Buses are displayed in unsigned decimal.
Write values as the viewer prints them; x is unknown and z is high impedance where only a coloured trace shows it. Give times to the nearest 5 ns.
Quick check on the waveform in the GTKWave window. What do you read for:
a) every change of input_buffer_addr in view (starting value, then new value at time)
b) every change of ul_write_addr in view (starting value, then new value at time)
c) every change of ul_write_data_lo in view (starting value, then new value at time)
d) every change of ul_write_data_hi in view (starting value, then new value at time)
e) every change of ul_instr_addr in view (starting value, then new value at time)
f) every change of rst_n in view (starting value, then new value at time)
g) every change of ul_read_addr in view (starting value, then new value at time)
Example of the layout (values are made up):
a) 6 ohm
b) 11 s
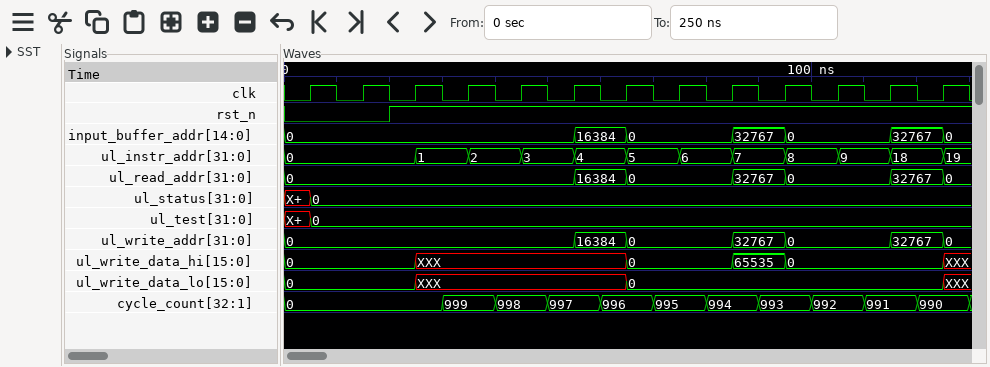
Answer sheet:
a) 0, 16384 at 55 ns, 0 at 65 ns, 32767 at 85 ns, 0 at 95 ns, 32767 at 115 ns, 0 at 125 ns
b) 0, 16384 at 55 ns, 0 at 65 ns, 32767 at 85 ns, 0 at 95 ns, 32767 at 115 ns, 0 at 125 ns
c) 0, XXX at 25 ns, 0 at 65 ns, XXX at 125 ns
d) 0, XXX at 25 ns, 0 at 65 ns, 65535 at 85 ns, 0 at 95 ns, XXX at 125 ns
e) 0, 1 at 25 ns, 2 at 35 ns, 3 at 45 ns, 4 at 55 ns, 5 at 65 ns, 6 at 75 ns, 7 at 85 ns, 8 at 95 ns, 9 at 105 ns, 18 at 115 ns, 19 at 125 ns
f) 0, 1 at 20 ns
g) 0, 16384 at 55 ns, 0 at 65 ns, 32767 at 85 ns, 0 at 95 ns, 32767 at 115 ns, 0 at 125 ns
